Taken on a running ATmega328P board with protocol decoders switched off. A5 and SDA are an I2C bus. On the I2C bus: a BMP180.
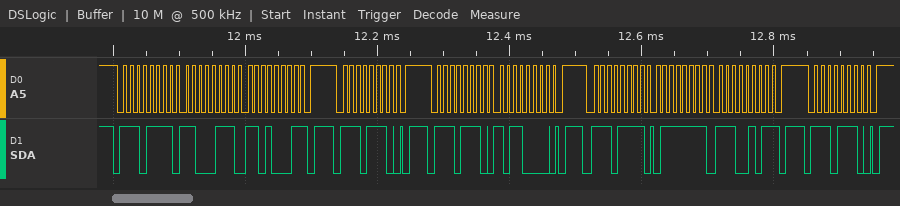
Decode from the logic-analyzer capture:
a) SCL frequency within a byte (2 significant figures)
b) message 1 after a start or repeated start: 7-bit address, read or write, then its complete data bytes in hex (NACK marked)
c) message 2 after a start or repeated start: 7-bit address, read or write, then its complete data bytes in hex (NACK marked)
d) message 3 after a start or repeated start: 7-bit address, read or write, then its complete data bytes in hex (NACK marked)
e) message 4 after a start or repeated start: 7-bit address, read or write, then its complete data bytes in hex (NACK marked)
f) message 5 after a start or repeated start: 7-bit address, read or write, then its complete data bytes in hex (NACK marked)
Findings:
100 kHz
0x77 read: C7 D1 NACK
0x77 write
0x77 write: B0
0x77 read: 7F E5 NACK
0x77 write
